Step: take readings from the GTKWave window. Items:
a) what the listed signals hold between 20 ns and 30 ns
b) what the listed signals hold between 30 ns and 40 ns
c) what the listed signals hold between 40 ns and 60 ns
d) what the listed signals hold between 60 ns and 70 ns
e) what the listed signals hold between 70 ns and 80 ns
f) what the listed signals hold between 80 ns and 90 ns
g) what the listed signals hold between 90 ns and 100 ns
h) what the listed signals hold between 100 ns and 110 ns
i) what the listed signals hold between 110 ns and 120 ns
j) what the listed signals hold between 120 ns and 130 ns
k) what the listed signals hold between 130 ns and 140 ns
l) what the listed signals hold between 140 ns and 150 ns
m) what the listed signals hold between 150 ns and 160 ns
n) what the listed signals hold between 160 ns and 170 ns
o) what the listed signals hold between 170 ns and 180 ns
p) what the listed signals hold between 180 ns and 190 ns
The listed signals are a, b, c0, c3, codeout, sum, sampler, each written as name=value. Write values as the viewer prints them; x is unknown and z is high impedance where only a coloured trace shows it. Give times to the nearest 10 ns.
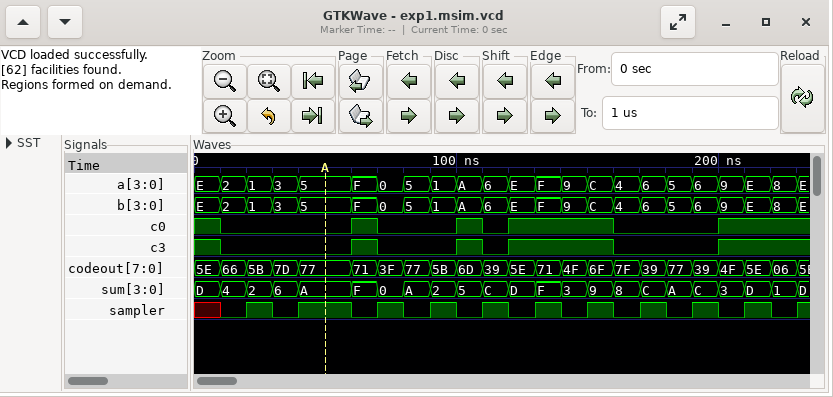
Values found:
a=1, b=1, c0=0, c3=0, codeout=5B, sum=2, sampler=1
a=3, b=3, c0=0, c3=0, codeout=7D, sum=6, sampler=0
a=5, b=5, c0=0, c3=0, codeout=77, sum=A, sampler=1
a=F, b=F, c0=1, c3=1, codeout=71, sum=F, sampler=0
a=0, b=0, c0=0, c3=0, codeout=3F, sum=0, sampler=1
a=5, b=5, c0=0, c3=0, codeout=77, sum=A, sampler=0
a=1, b=1, c0=0, c3=0, codeout=5B, sum=2, sampler=1
a=A, b=A, c0=1, c3=1, codeout=6D, sum=5, sampler=0
a=6, b=6, c0=0, c3=0, codeout=39, sum=C, sampler=1
a=E, b=E, c0=1, c3=1, codeout=5E, sum=D, sampler=0
a=F, b=F, c0=1, c3=1, codeout=71, sum=F, sampler=1
a=9, b=9, c0=1, c3=1, codeout=4F, sum=3, sampler=0
a=C, b=C, c0=1, c3=1, codeout=6F, sum=9, sampler=1
a=4, b=4, c0=0, c3=0, codeout=7F, sum=8, sampler=0
a=6, b=6, c0=0, c3=0, codeout=39, sum=C, sampler=1
a=5, b=5, c0=0, c3=0, codeout=77, sum=A, sampler=0
